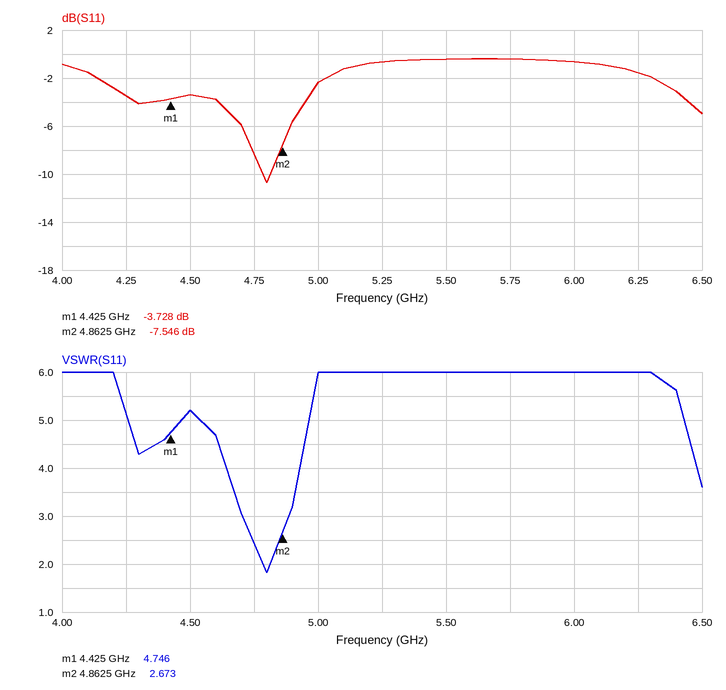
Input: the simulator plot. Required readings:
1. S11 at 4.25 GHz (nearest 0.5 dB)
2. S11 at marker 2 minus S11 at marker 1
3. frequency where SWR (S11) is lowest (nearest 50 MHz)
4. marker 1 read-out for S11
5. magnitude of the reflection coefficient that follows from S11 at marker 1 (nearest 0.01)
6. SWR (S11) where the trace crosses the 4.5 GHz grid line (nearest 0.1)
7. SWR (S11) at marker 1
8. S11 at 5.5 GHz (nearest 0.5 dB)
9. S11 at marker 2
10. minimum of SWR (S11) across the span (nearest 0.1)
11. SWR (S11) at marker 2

-3.5 dB
-3.818 dB
4.80 GHz
-3.728 dB
0.65
5.2
4.746
-0.5 dB
-7.546 dB
1.8
2.673
